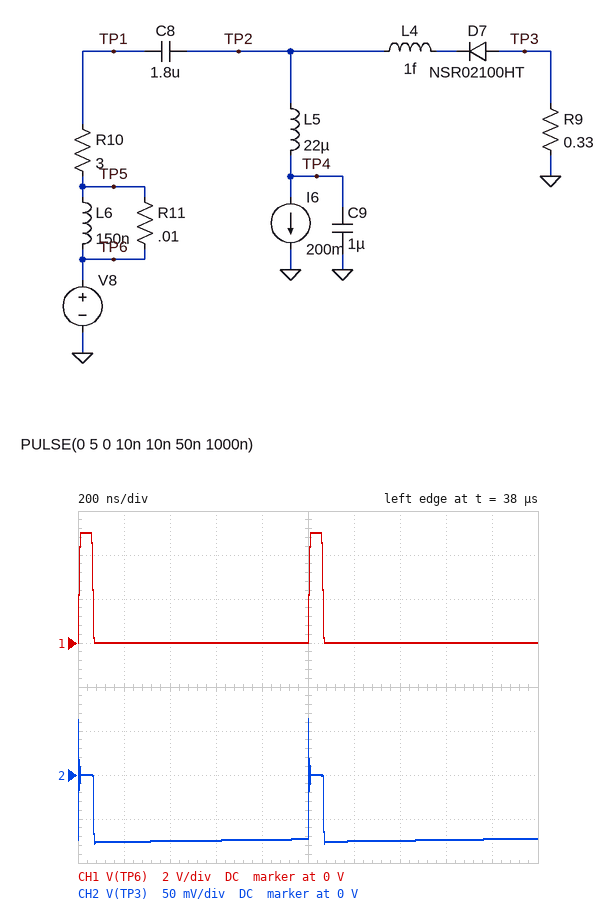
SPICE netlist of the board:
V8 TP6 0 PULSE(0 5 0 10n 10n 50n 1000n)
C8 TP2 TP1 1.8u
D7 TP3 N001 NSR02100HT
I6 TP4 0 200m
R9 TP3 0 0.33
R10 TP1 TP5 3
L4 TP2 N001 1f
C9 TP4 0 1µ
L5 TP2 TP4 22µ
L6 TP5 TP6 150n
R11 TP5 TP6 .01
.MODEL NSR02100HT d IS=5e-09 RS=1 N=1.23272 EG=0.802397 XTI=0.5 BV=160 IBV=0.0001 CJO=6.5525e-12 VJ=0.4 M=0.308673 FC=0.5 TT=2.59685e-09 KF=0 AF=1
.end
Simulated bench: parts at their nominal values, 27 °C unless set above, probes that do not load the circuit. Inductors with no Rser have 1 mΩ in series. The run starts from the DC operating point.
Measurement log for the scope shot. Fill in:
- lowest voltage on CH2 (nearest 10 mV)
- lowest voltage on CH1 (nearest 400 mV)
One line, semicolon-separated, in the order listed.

-80 mV; 0 V
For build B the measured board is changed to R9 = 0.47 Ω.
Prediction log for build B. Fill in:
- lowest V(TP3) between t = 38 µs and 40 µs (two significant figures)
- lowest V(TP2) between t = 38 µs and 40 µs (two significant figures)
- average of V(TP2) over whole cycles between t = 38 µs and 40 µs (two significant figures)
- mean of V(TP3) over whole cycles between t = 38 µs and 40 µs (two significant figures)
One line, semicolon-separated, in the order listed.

-110 mV; -900 mV; -640 mV; -98 mV
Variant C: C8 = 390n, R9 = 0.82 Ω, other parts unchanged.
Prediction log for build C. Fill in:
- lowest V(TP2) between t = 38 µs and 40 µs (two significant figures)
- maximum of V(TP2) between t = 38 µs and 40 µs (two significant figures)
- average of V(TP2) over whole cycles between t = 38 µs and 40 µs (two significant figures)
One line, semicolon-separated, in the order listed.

-980 mV; 3.4 V; -710 mV
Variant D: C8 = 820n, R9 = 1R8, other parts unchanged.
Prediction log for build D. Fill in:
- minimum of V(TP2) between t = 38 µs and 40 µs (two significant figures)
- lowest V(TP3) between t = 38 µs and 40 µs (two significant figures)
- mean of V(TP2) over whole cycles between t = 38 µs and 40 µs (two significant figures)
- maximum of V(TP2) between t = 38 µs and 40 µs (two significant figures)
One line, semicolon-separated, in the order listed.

-1.2 V; -410 mV; -910 mV; 3.2 V
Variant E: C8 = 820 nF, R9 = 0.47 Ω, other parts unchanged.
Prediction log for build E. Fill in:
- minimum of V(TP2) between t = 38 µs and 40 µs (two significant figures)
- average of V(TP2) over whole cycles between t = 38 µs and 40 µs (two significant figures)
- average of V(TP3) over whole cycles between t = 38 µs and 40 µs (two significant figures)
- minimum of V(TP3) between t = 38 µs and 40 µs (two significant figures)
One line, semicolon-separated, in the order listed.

-900 mV; -640 mV; -98 mV; -110 mV
